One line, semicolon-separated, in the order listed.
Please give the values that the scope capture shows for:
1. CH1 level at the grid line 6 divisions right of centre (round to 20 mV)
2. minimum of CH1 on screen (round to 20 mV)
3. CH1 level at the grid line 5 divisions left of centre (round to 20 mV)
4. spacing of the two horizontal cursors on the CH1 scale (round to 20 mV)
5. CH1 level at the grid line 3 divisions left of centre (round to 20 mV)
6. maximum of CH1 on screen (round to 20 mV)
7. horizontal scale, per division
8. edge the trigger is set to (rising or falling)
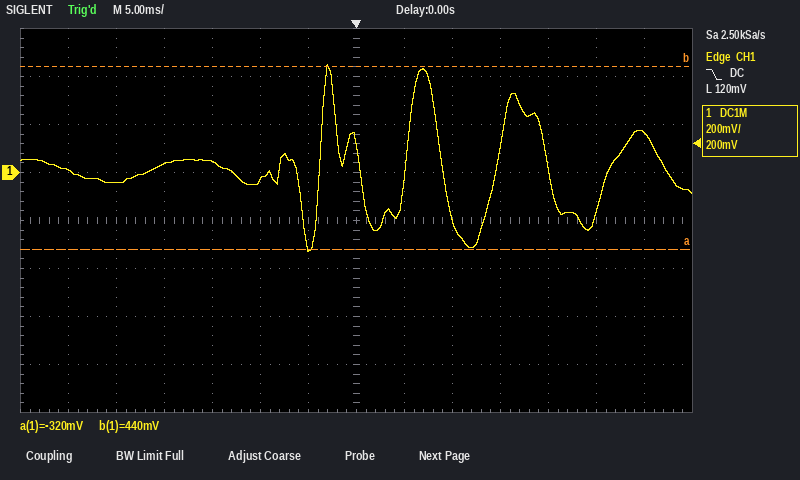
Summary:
160 mV; -320 mV; -40 mV; 760 mV; 40 mV; 440 mV; 5 ms; falling
